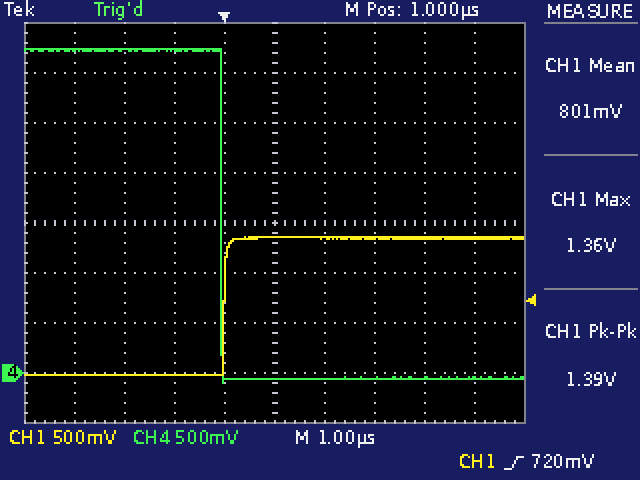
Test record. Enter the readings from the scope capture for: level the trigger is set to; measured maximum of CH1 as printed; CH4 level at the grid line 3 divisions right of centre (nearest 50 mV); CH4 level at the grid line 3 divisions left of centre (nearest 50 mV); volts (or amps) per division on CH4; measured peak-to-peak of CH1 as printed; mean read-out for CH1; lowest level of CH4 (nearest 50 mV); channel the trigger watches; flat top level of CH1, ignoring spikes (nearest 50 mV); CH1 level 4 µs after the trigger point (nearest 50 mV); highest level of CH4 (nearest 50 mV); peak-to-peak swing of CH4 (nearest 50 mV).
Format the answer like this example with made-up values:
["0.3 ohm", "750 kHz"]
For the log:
["720 mV", "1.36 V", "-50 mV", "3.25 V", "500 mV", "1.39 V", "801 mV", "-100 mV", "CH1", "1.35 V", "1.35 V", "3.25 V", "3.35 V"]
